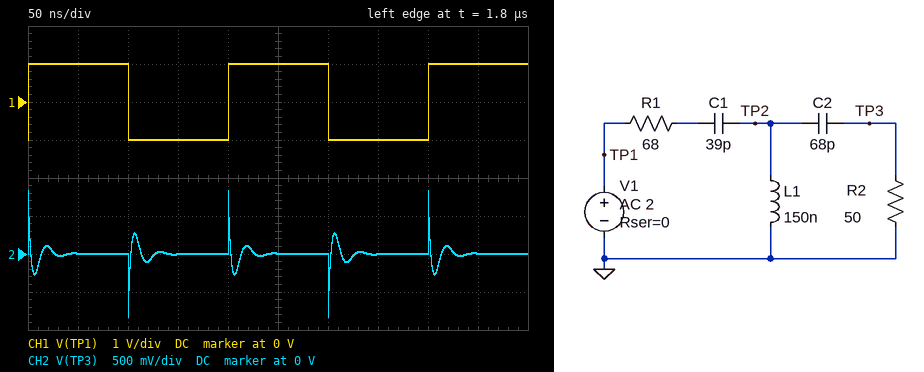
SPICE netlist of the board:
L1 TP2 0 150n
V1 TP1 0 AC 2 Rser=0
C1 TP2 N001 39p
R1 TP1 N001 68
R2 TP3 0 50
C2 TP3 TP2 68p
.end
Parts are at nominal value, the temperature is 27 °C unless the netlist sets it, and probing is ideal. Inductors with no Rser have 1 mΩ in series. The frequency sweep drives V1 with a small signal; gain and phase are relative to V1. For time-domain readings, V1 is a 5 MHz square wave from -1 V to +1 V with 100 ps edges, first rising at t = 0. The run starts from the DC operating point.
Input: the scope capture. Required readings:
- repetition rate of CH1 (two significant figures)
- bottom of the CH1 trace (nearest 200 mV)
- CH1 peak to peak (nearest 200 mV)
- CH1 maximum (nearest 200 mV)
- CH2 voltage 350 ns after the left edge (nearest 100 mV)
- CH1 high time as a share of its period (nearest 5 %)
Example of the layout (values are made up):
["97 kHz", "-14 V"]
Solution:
["5.0 MHz", "-1.0 V", "2.0 V", "1.0 V", "0 V", "50 %"]
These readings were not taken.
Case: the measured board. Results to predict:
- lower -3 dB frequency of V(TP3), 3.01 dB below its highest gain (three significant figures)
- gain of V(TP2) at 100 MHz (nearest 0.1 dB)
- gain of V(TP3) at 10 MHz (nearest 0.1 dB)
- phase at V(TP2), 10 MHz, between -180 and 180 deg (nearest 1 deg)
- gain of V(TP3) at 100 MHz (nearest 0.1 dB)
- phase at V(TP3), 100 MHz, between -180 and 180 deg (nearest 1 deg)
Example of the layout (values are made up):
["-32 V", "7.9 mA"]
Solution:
["38.2 MHz", "-6.8 dB", "-45.9 dB", "170 deg", "-7.6 dB", "49 deg"]
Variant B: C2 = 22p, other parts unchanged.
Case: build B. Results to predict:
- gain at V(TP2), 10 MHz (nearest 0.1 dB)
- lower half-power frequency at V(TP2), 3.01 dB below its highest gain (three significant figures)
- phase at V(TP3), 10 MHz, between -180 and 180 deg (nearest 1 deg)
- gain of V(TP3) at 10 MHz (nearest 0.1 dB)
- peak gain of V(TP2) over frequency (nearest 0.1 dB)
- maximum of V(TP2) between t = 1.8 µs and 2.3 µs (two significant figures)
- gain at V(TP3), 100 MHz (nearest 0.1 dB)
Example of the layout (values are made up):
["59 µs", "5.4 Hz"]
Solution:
["-32.5 dB", "45.0 MHz", "-104 deg", "-55.8 dB", "-0.3 dB", "860 mV", "-8.0 dB"]
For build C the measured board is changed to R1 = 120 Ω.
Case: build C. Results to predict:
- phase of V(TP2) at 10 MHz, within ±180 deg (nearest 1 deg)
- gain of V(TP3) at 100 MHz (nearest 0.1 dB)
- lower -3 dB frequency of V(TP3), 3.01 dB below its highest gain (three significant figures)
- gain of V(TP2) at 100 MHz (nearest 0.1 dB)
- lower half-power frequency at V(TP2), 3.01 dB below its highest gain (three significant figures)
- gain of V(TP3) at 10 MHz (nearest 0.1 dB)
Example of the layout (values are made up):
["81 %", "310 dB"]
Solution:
["163 deg", "-10.5 dB", "38.5 MHz", "-9.6 dB", "33.1 MHz", "-46.2 dB"]
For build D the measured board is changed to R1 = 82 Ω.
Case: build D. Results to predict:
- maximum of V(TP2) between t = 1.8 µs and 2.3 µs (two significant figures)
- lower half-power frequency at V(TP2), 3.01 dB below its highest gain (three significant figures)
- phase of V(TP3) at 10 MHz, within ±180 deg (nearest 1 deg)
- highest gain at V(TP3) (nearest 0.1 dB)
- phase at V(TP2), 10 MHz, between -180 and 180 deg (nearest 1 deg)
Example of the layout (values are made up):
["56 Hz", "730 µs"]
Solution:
["750 mV", "33.6 MHz", "-114 deg", "-8.4 dB", "168 deg"]
